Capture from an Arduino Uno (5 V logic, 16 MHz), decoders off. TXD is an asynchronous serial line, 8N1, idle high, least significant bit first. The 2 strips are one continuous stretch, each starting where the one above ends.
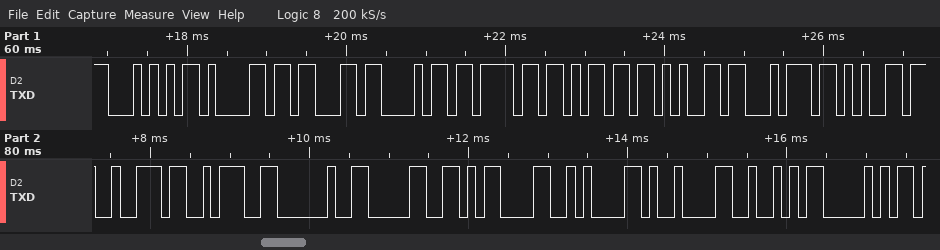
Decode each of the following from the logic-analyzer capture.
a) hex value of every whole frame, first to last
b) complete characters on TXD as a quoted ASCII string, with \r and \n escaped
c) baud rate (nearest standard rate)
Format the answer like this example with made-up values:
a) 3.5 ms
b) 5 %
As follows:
a) 54 61 63 68 6F 6D 65 74 65 72 3A 20 30 0D 0A 09 52 50
b) "Tachometer: 0\r\n\tRP"
c) 9600 baud
